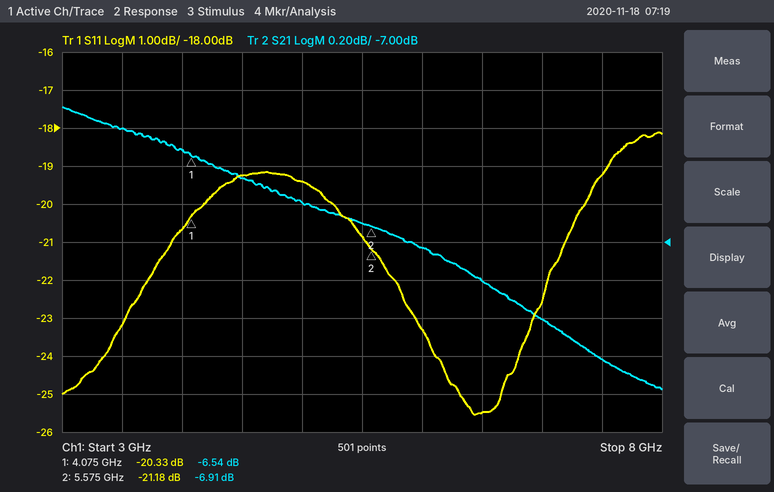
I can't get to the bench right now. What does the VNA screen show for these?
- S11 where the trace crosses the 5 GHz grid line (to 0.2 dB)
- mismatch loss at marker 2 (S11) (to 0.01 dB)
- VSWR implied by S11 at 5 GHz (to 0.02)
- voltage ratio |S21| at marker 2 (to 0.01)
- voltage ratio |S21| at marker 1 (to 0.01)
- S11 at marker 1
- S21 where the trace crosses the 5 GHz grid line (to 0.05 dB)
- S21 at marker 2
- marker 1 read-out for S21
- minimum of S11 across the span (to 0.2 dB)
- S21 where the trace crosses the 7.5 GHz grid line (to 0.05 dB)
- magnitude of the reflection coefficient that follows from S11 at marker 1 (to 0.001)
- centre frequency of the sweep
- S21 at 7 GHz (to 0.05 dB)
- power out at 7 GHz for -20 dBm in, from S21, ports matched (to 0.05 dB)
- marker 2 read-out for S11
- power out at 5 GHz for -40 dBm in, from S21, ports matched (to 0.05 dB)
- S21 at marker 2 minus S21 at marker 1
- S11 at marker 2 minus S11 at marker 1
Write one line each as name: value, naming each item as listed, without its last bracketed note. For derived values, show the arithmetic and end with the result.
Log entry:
S11 where the trace crosses the 5 GHz grid line: -19.4 dB
mismatch loss at marker 2 (S11): −10 log10(1 − 10^(-21.18/10)) ≈ 0.03 dB
VSWR implied by S11 at 5 GHz: |Γ| = 10^(-19.4/20) = 0.1072; VSWR = (1 + 0.1072)/(1 − 0.1072) ≈ 1.24
voltage ratio |S21| at marker 2: 10^(-6.91/20) ≈ 0.45
voltage ratio |S21| at marker 1: 10^(-6.54/20) ≈ 0.47
S11 at marker 1: -20.33 dB
S21 where the trace crosses the 5 GHz grid line: -6.80 dB
S21 at marker 2: -6.91 dB
marker 1 read-out for S21: -6.54 dB
minimum of S11 across the span: -25.6 dB
S21 where the trace crosses the 7.5 GHz grid line: -7.60 dB
magnitude of the reflection coefficient that follows from S11 at marker 1: 10^(-20.33/20) ≈ 0.096
centre frequency of the sweep: 5.5 GHz
S21 at 7 GHz: -7.40 dB
power out at 7 GHz for -20 dBm in, from S21, ports matched: -20 dBm + (-7.40 dB) = -27.40 dBm
marker 2 read-out for S11: -21.18 dB
power out at 5 GHz for -40 dBm in, from S21, ports matched: -40 dBm + (-6.80 dB) = -46.80 dBm
S21 at marker 2 minus S21 at marker 1: -6.91 − (-6.54) = -0.37 dB
S11 at marker 2 minus S11 at marker 1: -21.18 − (-20.33) = -0.85 dB
